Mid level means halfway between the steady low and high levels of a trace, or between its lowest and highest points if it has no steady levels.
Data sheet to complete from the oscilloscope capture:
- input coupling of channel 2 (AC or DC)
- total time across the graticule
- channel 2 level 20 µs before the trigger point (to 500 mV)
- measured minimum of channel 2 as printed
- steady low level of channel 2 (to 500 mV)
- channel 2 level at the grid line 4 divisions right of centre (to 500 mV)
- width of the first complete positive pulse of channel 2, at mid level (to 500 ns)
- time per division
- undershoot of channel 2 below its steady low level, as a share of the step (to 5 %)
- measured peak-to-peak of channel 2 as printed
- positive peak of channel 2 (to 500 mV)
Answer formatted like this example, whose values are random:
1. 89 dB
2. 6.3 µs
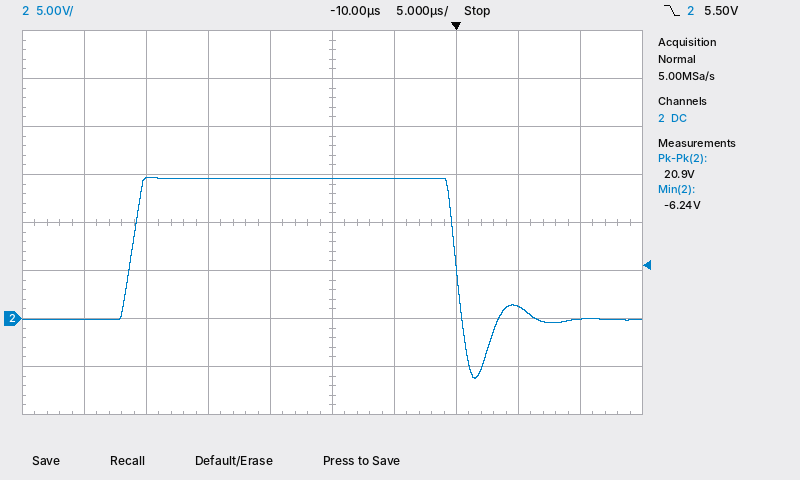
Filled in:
1. DC
2. 50 µs
3. 14.5 V
4. -6.24 V
5. 0.0 V
6. 0.0 V
7. 26.0 µs
8. 5 µs
9. 40 %
10. 20.9 V
11. 14.5 V
